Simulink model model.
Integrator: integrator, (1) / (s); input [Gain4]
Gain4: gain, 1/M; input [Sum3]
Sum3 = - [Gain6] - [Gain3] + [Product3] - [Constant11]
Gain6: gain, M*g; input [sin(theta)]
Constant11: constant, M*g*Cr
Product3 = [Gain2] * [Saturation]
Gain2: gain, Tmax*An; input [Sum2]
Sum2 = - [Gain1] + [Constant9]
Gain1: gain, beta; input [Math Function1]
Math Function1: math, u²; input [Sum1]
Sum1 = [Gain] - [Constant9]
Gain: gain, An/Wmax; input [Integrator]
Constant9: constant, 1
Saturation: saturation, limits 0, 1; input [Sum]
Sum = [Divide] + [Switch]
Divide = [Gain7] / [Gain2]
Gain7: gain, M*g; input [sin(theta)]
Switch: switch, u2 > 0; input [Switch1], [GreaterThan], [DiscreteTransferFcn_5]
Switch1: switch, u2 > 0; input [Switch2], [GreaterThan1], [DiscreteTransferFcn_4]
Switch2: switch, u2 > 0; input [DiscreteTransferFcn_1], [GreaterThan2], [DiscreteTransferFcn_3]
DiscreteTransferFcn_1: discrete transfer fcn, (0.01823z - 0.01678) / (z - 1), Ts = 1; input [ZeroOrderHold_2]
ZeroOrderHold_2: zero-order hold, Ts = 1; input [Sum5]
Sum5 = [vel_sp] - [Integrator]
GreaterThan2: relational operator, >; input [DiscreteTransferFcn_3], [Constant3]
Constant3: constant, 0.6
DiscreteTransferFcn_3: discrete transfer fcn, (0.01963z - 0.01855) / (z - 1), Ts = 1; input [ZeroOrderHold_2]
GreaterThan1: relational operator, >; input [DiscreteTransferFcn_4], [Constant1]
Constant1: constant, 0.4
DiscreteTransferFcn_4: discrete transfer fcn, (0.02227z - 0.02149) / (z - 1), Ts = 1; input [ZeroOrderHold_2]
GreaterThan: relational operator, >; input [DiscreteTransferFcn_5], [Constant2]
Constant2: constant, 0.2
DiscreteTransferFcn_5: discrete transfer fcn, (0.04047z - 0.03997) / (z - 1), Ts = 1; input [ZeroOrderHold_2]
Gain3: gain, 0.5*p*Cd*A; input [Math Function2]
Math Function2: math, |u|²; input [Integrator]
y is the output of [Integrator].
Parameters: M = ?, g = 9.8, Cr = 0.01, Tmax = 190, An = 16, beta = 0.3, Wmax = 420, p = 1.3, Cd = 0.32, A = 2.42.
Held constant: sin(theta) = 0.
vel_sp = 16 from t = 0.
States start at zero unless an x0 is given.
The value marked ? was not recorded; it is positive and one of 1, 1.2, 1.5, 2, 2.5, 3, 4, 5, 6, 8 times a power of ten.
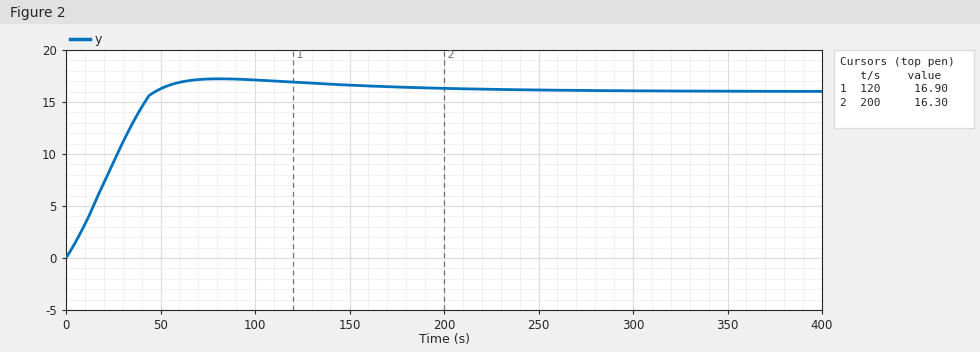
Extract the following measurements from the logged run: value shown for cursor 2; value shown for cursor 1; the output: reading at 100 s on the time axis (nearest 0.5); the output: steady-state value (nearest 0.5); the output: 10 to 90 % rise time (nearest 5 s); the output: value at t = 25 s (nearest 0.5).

16.30
16.90
17.0
16.0
35 s
9.0
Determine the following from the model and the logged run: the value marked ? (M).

2000
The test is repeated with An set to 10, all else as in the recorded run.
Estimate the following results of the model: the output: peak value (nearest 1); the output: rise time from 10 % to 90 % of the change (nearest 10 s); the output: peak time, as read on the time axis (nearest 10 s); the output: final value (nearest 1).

17
40 s
60 s
16
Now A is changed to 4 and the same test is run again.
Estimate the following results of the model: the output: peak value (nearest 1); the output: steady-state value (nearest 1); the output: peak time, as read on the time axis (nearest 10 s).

17
16
80 s
